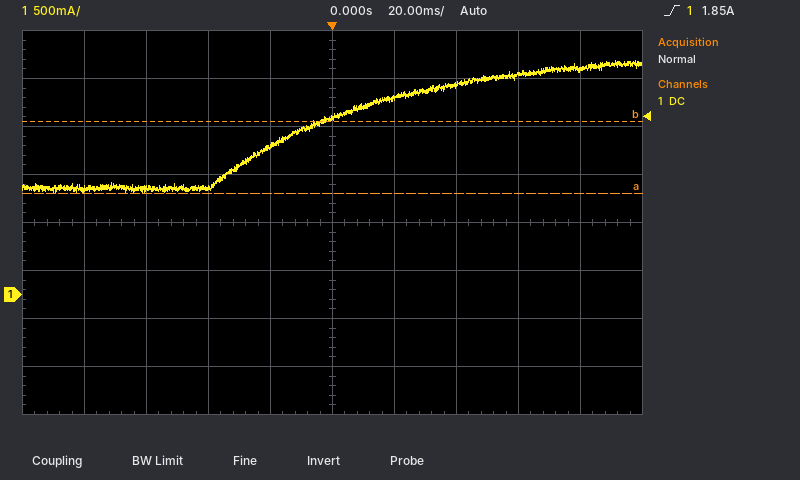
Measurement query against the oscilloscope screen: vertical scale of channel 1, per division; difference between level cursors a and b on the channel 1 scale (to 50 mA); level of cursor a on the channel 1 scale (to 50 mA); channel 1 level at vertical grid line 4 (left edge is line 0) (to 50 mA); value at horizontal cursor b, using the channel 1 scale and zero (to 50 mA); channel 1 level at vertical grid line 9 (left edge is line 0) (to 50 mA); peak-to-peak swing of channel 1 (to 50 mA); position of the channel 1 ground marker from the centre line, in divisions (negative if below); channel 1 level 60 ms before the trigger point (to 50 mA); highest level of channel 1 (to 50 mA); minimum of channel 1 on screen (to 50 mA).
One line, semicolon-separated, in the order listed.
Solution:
500 mA; 750 mA; 1.05 A; 1.55 A; 1.80 A; 2.35 A; 1.40 A; -1.5 div; 1.10 A; 2.45 A; 1.05 A
